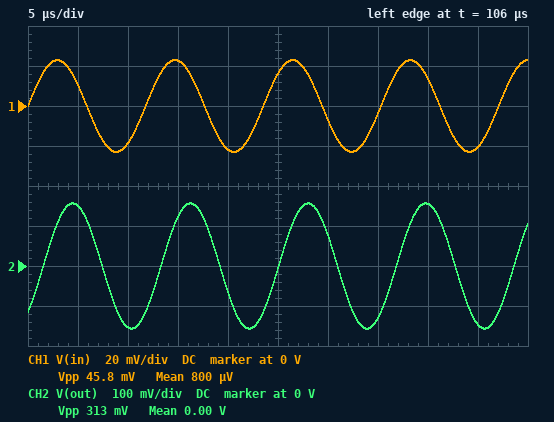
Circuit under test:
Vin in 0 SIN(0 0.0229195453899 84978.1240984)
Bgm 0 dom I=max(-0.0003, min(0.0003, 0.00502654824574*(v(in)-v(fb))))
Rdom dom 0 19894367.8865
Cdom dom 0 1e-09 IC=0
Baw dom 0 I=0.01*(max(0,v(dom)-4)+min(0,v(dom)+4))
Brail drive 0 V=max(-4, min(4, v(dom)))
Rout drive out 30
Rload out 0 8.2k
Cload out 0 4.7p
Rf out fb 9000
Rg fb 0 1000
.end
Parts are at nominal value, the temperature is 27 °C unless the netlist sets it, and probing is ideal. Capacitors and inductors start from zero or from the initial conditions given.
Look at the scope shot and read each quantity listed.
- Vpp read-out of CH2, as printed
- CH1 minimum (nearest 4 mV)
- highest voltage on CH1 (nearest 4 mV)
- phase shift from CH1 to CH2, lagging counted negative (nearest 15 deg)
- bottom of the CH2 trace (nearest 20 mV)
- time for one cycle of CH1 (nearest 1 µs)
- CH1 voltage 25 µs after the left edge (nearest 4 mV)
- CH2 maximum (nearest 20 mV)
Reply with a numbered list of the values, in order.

1. 313 mV
2. -24 mV
3. 24 mV
4. -45 deg
5. -160 mV
6. 12 µs
7. 16 mV
8. 160 mV
